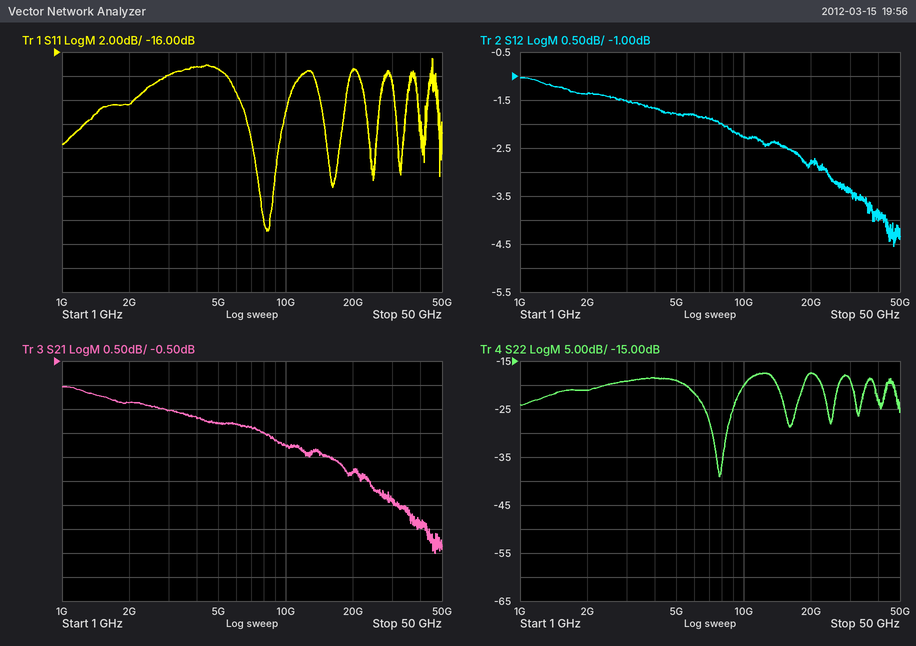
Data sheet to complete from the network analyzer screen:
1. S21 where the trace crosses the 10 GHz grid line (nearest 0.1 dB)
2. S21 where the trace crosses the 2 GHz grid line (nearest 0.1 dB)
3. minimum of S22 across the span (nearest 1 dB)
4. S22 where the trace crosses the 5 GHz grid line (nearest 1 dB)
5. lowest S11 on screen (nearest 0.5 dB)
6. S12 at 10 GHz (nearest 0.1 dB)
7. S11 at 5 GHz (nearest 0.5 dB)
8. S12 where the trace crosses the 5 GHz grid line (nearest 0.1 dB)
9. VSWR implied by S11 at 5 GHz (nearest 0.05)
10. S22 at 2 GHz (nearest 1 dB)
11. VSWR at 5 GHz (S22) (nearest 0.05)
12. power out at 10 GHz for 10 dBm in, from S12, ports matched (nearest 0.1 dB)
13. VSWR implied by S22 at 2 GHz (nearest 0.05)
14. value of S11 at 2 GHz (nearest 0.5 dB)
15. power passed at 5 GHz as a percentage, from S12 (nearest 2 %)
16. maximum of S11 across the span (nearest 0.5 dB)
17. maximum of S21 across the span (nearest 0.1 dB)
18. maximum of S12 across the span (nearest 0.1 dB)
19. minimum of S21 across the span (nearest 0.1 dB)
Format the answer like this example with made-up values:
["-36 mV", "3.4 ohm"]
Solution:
["-2.3 dB", "-1.4 dB", "-39 dB", "-19 dB", "-31.0 dB", "-2.3 dB", "-17.5 dB", "-1.8 dB", "1.30", "-21 dB", "1.25", "7.7 dBm", "1.20", "-20.5 dB", "66 %", "-16.5 dB", "-1.0 dB", "-1.0 dB", "-4.5 dB"]
